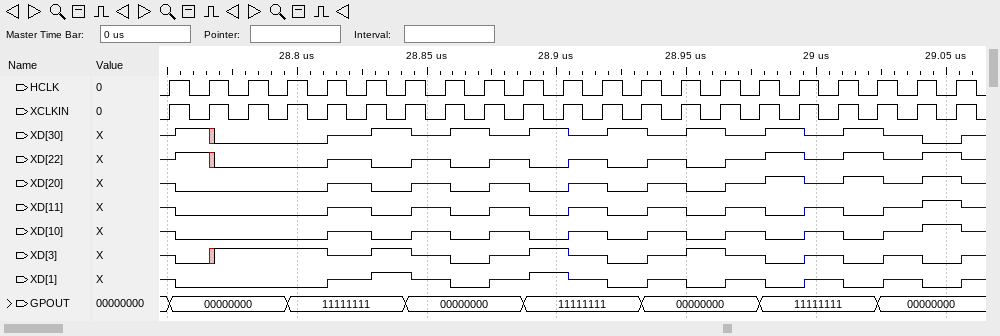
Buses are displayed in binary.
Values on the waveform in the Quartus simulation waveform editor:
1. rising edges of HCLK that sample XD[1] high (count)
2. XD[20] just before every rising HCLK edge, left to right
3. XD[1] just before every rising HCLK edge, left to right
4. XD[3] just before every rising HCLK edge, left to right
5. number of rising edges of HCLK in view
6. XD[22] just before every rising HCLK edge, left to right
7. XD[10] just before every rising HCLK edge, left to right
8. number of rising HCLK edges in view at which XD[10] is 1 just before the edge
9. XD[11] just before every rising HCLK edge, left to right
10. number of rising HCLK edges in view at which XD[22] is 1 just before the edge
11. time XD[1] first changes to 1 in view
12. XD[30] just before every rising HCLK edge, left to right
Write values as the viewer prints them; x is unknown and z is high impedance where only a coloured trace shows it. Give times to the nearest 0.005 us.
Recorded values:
2
z 0 0 0 0 z 0 z 0 z 0 z 0 z 0 z 1 z 1 z 1
z 0 0 0 0 z 1 z 0 z 1 z 0 z 0 z 0 z 0 z 0
z 0 1 1 1 z 1 z 0 z 1 z 0 z 1 z 0 z 0 z 0
21
z 1 0 0 0 z 0 z 0 z 0 z 0 z 0 z 1 z 1 z 1
z 0 0 0 0 z 0 z 0 z 0 z 0 z 0 z 0 z 0 z 1
1
z 0 0 0 0 z 0 z 0 z 0 z 0 z 0 z 0 z 0 z 1
4
28.83 us
z 1 0 0 0 z 1 z 1 z 1 z 1 z 1 z 1 z 1 z 0
